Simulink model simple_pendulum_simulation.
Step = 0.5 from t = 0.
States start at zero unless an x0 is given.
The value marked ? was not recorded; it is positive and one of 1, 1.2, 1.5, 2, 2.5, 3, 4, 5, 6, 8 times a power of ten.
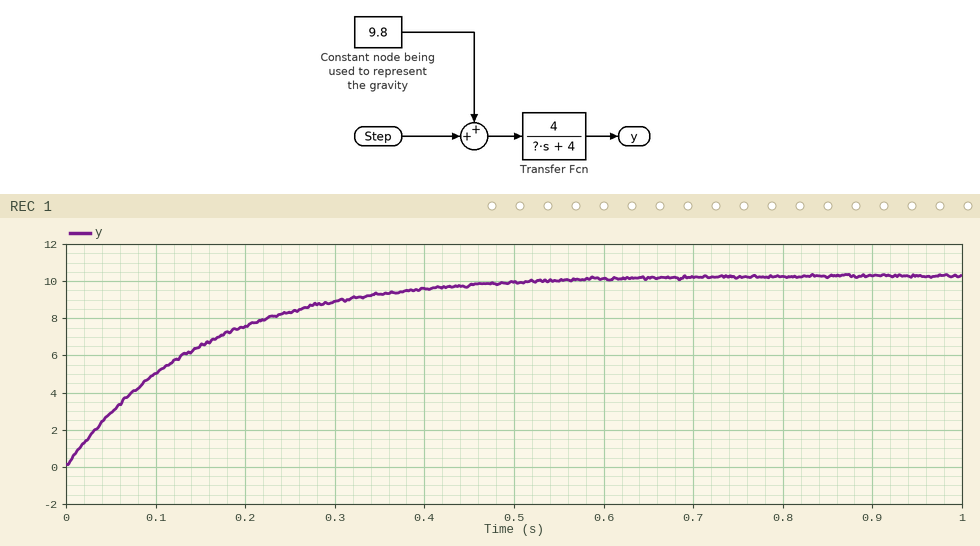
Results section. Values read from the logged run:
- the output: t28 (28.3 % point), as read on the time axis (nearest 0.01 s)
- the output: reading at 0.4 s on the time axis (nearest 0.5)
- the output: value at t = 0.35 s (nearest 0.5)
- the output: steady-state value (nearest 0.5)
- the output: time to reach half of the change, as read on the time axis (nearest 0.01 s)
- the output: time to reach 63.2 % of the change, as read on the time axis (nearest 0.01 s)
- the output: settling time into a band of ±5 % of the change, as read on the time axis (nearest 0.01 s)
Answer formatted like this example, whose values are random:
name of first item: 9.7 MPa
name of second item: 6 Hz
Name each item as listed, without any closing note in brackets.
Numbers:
the output: t28 (28.3 % point), as read on the time axis: 0.05 s
the output: reading at 0.4 s on the time axis: 9.5
the output: value at t = 0.35 s: 9.5
the output: steady-state value: 10.5
the output: time to reach half of the change, as read on the time axis: 0.10 s
the output: time to reach 63.2 % of the change, as read on the time axis: 0.15 s
the output: settling time into a band of ±5 % of the change, as read on the time axis: 0.45 s
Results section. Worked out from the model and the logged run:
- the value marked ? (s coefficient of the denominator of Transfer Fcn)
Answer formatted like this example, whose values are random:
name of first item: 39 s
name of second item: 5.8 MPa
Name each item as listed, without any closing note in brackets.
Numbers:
the value marked ?: 0.6
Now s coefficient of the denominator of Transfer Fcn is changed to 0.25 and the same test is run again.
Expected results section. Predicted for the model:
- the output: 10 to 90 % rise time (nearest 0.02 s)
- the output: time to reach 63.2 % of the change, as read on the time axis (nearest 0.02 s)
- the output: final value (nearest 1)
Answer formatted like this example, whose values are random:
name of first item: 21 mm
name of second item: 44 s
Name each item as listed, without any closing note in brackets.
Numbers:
the output: 10 to 90 % rise time: 0.14 s
the output: time to reach 63.2 % of the change, as read on the time axis: 0.06 s
the output: final value: 10
